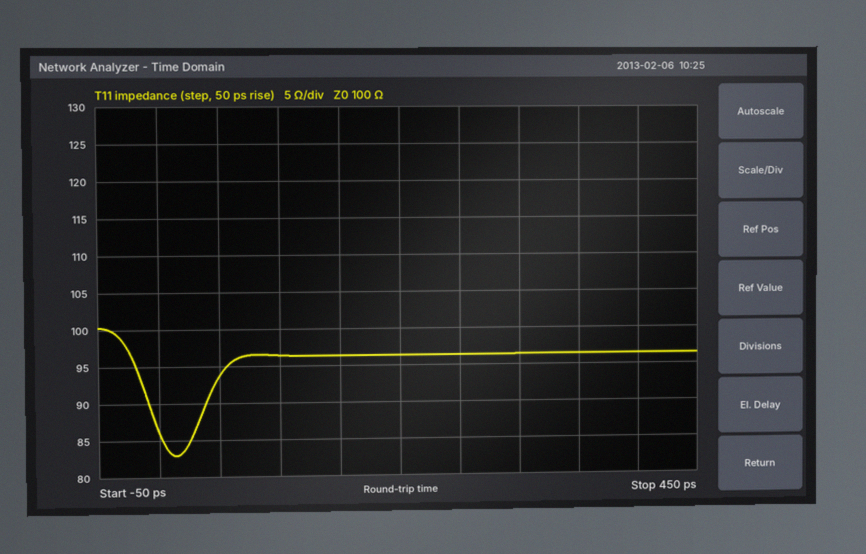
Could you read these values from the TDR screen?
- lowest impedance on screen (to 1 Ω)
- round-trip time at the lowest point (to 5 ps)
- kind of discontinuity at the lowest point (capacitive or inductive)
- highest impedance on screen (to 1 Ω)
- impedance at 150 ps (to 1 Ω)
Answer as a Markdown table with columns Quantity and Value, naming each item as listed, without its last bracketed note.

| Quantity | Value |
|---|---|
| lowest impedance on screen | 83 Ω |
| round-trip time at the lowest point | 15 ps |
| kind of discontinuity at the lowest point | capacitive |
| highest impedance on screen | 100 Ω |
| impedance at 150 ps | 96 Ω |
